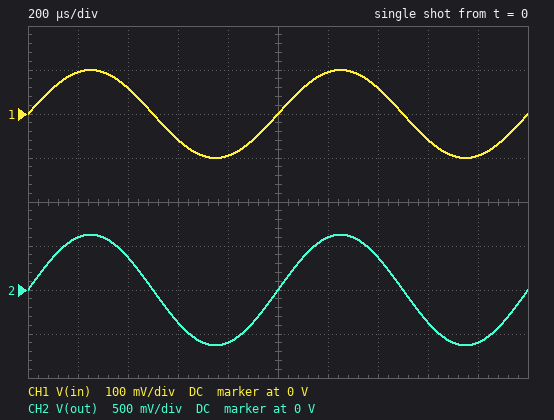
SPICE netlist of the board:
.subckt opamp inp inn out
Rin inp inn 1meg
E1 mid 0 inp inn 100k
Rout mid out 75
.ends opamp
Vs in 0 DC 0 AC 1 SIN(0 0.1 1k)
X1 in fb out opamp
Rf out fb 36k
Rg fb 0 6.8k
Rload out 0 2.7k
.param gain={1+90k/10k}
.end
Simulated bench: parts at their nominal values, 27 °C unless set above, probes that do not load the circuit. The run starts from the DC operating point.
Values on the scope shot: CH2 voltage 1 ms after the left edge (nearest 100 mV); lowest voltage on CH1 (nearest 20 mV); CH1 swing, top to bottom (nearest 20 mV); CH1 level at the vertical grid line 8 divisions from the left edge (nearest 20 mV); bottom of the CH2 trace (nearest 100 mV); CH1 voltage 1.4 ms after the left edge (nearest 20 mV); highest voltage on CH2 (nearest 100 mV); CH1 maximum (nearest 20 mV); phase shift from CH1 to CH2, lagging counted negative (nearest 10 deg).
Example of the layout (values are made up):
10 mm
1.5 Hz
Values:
0 V
-100 mV
200 mV
-60 mV
-600 mV
60 mV
600 mV
100 mV
0 deg
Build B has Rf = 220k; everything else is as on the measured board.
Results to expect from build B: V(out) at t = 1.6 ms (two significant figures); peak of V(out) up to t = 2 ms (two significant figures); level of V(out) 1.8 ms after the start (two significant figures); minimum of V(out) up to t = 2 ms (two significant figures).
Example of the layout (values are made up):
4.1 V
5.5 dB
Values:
-2.0 V
3.3 V
-3.2 V
-3.3 V
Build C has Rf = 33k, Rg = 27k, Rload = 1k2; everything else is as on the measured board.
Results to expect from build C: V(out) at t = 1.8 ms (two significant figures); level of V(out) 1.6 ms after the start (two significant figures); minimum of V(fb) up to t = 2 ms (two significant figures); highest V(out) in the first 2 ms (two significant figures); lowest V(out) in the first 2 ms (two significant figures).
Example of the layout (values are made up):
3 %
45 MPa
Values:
-210 mV
-130 mV
-100 mV
220 mV
-220 mV
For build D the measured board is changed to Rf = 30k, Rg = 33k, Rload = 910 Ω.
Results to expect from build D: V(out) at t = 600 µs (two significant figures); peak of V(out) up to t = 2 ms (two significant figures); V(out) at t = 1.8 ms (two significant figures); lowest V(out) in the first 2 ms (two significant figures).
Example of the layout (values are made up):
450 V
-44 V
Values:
-110 mV
190 mV
-180 mV
-190 mV
